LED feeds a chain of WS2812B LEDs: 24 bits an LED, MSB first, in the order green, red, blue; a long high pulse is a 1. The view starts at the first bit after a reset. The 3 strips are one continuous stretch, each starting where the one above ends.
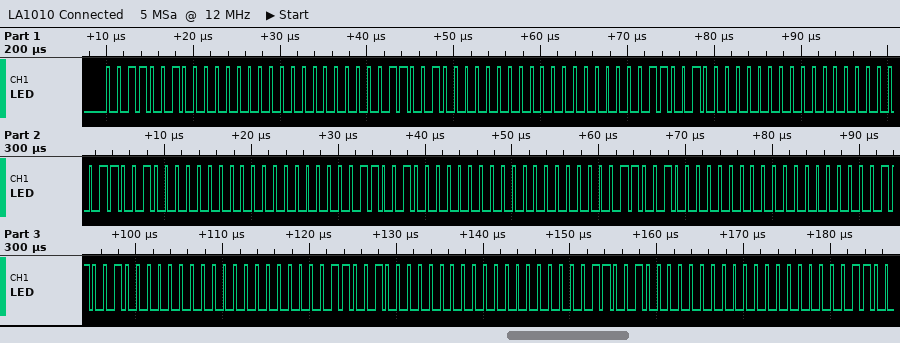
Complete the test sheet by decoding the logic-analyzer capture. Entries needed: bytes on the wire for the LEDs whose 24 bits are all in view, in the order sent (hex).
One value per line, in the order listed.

32 00 00 32 00 00 32 00 00 32 00 00 32 00 00 32 00 00 32 00 00 32 00 00 32 00 00
